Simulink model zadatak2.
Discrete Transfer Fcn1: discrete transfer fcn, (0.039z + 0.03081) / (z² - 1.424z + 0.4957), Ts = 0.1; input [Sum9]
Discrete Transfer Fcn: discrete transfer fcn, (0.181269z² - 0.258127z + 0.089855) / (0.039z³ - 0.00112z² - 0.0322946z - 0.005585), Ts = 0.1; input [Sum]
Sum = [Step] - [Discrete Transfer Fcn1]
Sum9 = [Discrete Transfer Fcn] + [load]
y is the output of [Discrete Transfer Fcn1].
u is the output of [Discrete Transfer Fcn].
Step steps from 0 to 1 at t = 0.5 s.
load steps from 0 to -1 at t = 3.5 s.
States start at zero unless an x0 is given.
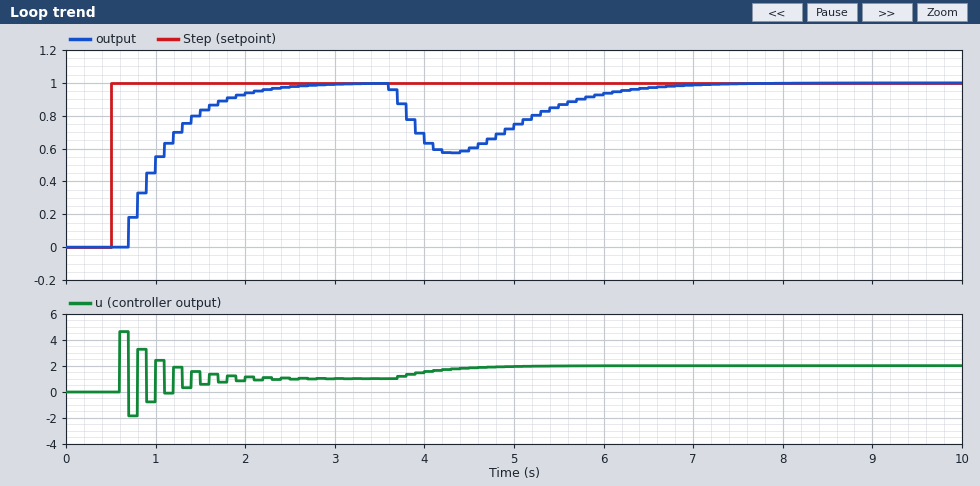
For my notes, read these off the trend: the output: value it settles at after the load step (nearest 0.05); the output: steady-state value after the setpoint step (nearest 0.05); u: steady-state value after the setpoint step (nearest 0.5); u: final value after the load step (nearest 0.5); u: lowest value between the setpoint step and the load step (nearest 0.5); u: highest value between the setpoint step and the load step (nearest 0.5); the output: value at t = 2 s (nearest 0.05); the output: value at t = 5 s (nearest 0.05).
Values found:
1.00
1.00
1.0
2.0
-2.0
4.5
0.95
0.75
